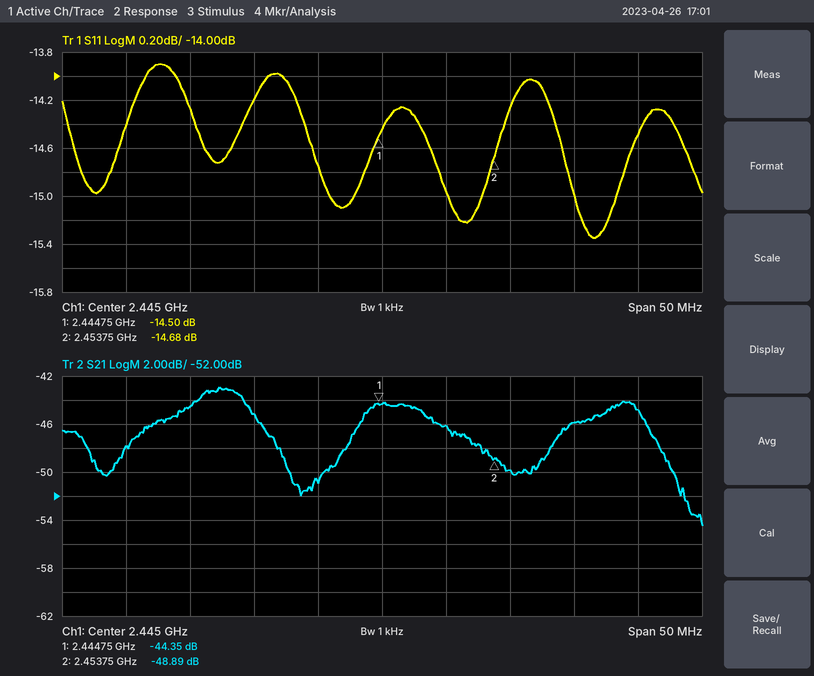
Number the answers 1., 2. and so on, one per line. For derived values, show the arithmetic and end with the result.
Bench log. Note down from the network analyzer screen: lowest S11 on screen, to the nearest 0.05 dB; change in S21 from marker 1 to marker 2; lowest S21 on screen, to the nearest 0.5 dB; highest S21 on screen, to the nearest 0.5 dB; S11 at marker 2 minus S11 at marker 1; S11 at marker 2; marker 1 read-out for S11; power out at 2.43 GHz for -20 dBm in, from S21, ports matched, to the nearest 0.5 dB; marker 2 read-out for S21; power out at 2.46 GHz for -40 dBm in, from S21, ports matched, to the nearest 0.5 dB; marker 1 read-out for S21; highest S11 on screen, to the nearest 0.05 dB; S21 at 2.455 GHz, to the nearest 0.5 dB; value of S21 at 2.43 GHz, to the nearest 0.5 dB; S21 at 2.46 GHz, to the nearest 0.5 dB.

1. -15.35 dB
2. -48.89 − (-44.35) = -4.54 dB
3. -54.5 dB
4. -43.0 dB
5. -14.68 − (-14.5) = -0.18 dB
6. -14.68 dB
7. -14.50 dB
8. -20 dBm + (-44.5 dB) = -64.5 dBm
9. -48.89 dB
10. -40 dBm + (-46.0 dB) = -86.0 dBm
11. -44.35 dB
12. -13.90 dB
13. -50.0 dB
14. -44.5 dB
15. -46.0 dB
